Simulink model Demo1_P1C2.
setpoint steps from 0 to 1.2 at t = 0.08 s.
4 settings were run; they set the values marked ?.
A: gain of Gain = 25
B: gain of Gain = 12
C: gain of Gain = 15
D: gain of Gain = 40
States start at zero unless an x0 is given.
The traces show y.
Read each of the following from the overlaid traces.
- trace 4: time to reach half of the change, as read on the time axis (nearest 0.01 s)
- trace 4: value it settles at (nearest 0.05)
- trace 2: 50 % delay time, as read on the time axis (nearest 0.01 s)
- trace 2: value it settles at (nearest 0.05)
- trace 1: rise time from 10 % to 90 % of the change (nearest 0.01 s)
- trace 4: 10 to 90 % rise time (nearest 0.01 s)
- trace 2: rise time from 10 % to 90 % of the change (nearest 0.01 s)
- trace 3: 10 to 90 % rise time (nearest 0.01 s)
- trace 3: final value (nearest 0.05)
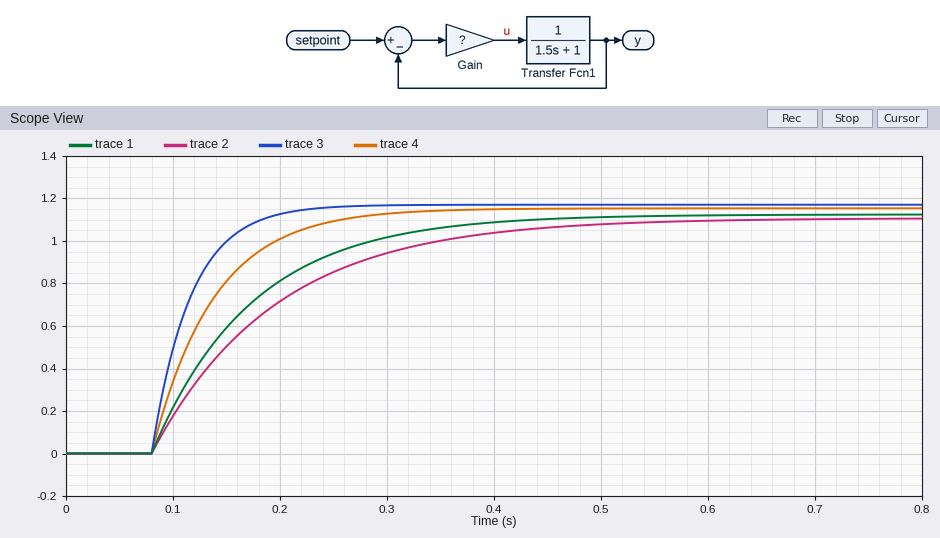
0.12 s
1.15
0.16 s
1.10
0.21 s
0.13 s
0.25 s
0.08 s
1.15
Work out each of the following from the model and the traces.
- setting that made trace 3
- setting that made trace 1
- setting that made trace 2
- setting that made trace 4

D
C
B
A
